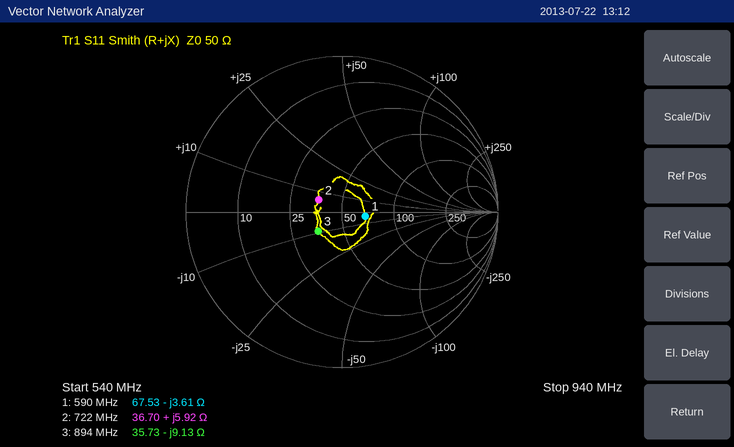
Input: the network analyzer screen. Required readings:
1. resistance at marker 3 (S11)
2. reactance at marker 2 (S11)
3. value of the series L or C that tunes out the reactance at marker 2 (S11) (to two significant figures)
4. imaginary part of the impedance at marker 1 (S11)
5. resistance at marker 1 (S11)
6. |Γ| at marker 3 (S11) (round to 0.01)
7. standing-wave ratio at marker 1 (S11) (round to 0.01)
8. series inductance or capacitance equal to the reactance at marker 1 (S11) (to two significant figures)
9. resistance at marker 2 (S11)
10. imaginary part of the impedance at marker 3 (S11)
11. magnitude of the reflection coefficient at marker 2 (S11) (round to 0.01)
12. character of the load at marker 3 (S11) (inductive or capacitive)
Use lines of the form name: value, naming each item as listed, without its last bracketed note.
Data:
resistance at marker 3: 35.73 Ω
reactance at marker 2: +5.92 Ω
value of the series L or C that tunes out the reactance at marker 2 (S11): 37 pF
imaginary part of the impedance at marker 1: -3.61 Ω
resistance at marker 1: 67.53 Ω
|Γ| at marker 3 (S11): 0.20
standing-wave ratio at marker 1 (S11): 1.36
series inductance or capacitance equal to the reactance at marker 1 (S11): 75 pF
resistance at marker 2: 36.70 Ω
imaginary part of the impedance at marker 3: -9.13 Ω
magnitude of the reflection coefficient at marker 2 (S11): 0.17
character of the load at marker 3 (S11): capacitive
